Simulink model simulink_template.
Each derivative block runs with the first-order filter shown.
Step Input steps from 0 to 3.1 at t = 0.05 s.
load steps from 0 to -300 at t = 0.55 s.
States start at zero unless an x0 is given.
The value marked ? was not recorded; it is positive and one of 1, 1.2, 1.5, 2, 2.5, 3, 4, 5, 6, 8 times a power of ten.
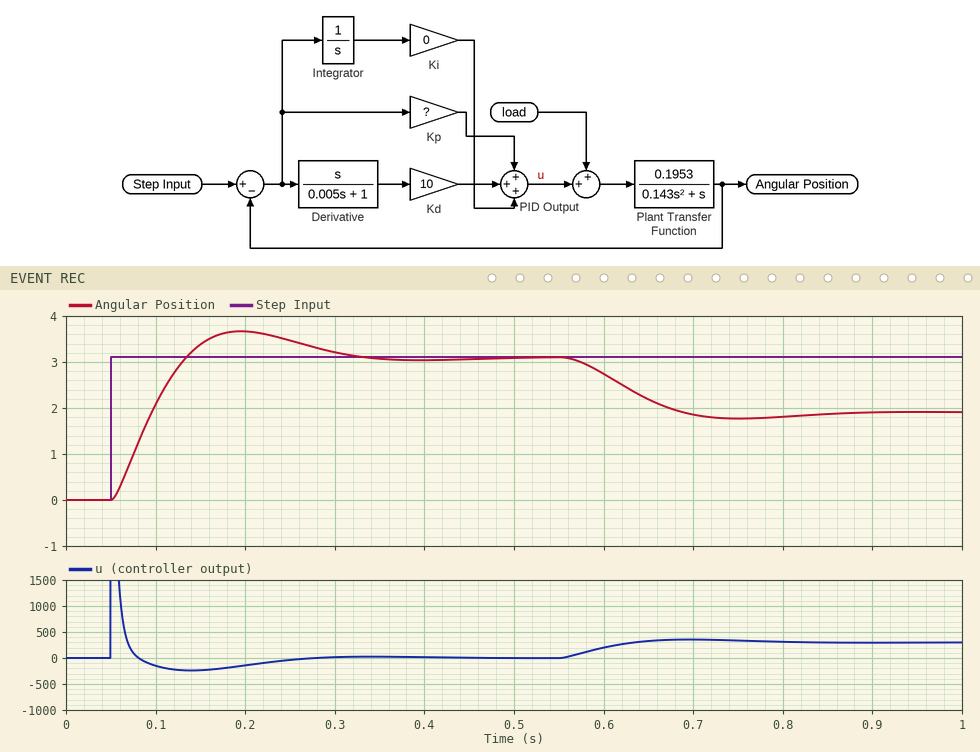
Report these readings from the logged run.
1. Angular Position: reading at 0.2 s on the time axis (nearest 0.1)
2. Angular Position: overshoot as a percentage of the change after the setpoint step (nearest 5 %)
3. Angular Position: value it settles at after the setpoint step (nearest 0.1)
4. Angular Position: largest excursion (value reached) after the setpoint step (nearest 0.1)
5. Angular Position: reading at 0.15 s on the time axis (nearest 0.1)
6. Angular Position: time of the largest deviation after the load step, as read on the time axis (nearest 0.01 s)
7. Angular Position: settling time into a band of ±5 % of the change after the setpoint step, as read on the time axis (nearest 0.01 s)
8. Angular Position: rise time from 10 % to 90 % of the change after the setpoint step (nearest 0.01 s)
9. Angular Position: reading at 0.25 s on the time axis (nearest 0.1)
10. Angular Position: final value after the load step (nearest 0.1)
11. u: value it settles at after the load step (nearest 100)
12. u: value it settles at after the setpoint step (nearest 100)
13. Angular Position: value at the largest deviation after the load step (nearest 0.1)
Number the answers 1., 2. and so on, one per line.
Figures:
1. 3.7
2. 20 %
3. 3.1
4. 3.7
5. 3.4
6. 0.75 s
7. 0.29 s
8. 0.06 s
9. 3.5
10. 1.9
11. 300
12. 0
13. 1.8
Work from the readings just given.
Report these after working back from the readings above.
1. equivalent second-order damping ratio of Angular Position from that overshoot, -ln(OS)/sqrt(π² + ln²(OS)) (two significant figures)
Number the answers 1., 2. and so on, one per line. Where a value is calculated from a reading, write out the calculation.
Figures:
1. ln(0.2) = -1.609; 1.609 / sqrt(9.870 + 2.590) = 0.46
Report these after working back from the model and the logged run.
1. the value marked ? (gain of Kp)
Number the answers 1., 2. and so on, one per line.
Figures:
1. 250
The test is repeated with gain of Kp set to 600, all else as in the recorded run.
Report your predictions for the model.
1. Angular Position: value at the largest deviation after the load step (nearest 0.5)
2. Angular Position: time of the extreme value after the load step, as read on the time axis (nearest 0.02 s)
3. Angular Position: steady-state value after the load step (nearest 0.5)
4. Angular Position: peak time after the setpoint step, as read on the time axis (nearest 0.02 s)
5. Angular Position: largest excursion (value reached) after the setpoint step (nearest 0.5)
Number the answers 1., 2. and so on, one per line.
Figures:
1. 2.5
2. 0.66 s
3. 2.5
4. 0.14 s
5. 4.0
